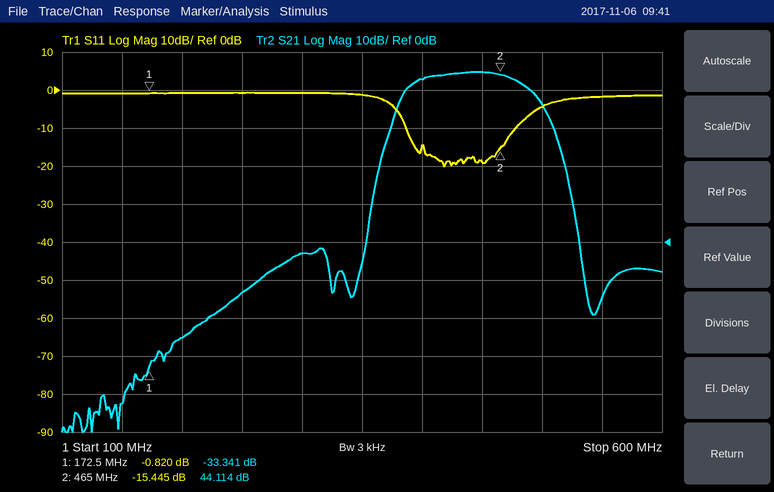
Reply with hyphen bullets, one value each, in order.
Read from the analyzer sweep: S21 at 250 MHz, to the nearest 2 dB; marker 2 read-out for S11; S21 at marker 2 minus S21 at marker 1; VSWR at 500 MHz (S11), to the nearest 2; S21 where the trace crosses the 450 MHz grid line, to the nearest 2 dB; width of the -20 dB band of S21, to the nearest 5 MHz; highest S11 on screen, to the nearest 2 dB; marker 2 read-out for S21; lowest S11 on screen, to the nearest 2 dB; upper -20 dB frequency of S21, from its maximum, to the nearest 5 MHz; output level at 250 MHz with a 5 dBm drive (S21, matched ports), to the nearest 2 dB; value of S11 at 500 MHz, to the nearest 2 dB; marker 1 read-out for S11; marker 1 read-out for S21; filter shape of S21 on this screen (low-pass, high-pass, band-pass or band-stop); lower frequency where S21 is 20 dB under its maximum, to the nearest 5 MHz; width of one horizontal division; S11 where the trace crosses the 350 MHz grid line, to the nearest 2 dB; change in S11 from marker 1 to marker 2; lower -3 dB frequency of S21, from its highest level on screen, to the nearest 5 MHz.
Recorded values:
- -14 dB
- -15.445 dB
- 77.455 dB
- 4
- 44 dB
- 145 MHz
- 0 dB
- 44.114 dB
- -20 dB
- 515 MHz
- -8 dBm
- -4 dB
- -0.820 dB
- -33.341 dB
- band-pass
- 370 MHz
- 50 MHz
- -2 dB
- -14.625 dB
- 395 MHz
